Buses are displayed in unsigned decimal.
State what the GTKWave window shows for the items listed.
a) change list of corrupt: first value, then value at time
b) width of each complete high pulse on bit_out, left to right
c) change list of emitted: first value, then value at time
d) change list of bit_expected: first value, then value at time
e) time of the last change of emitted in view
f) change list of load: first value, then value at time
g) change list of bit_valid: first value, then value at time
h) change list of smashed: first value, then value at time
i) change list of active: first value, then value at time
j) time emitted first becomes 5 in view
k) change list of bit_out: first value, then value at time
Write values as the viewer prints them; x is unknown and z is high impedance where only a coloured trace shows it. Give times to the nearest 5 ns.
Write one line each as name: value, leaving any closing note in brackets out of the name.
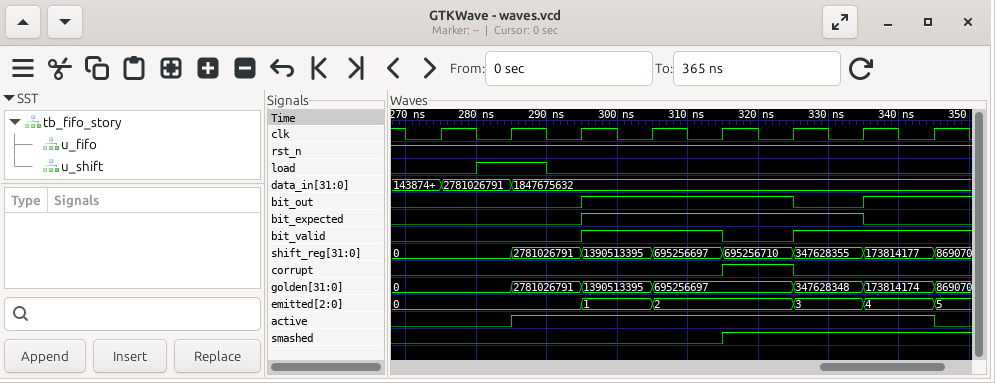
change list of corrupt: first value, then value at time: 0, 1 at 315 ns, 0 at 325 ns
width of each complete high pulse on bit_out, left to right: 30 ns
change list of emitted: first value, then value at time: 0, 1 at 295 ns, 2 at 305 ns, 3 at 325 ns, 4 at 335 ns, 5 at 345 ns
change list of bit_expected: first value, then value at time: 0, 1 at 295 ns, 0 at 335 ns
time of the last change of emitted in view: 345 ns
change list of load: first value, then value at time: 0, 1 at 280 ns, 0 at 290 ns
change list of bit_valid: first value, then value at time: 0, 1 at 295 ns, 0 at 315 ns, 1 at 325 ns
change list of smashed: first value, then value at time: 0, 1 at 315 ns
change list of active: first value, then value at time: 0, 1 at 285 ns, 0 at 345 ns
time emitted first becomes 5 in view: 345 ns
change list of bit_out: first value, then value at time: 0, 1 at 295 ns, 0 at 325 ns, 1 at 335 ns
